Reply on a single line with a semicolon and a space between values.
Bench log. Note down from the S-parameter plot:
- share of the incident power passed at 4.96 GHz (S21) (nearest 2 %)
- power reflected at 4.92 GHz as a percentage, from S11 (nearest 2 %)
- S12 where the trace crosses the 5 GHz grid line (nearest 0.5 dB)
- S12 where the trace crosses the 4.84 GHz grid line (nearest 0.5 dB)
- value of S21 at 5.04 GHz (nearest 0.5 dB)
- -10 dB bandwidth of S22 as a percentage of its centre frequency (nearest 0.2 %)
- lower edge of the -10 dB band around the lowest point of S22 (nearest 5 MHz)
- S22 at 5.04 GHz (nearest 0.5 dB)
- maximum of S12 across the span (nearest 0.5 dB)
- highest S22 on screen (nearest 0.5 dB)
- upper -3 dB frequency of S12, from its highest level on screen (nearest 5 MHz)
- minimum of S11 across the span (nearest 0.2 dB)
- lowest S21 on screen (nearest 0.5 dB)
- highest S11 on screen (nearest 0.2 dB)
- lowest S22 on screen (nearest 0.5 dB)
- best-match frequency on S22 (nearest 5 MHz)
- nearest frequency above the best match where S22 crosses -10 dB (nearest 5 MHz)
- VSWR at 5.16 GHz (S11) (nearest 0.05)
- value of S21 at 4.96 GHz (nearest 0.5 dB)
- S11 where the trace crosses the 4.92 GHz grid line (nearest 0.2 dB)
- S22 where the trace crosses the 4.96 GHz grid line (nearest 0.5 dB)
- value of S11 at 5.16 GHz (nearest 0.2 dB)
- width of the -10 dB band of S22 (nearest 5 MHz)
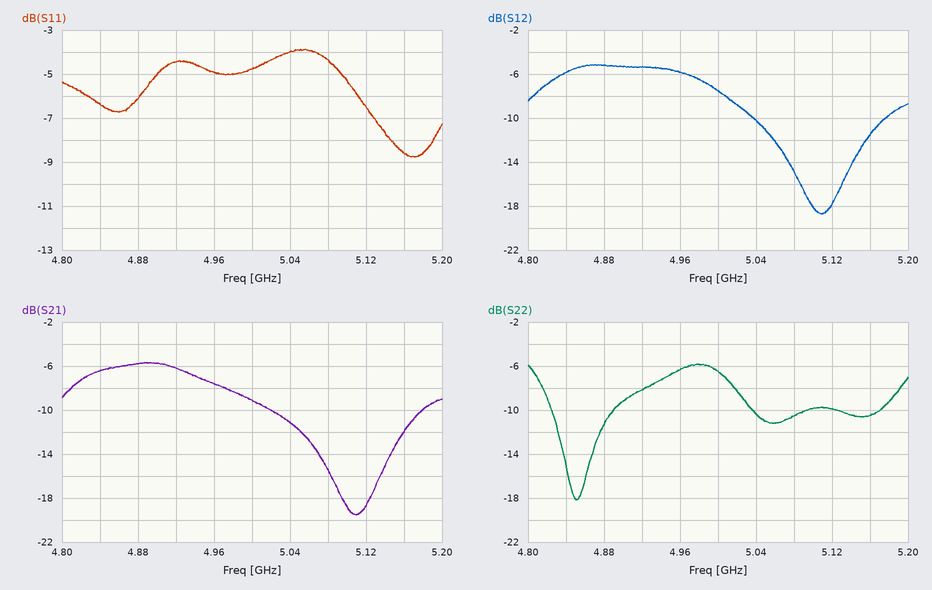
18 %; 36 %; -7.5 dB; -6.0 dB; -11.0 dB; 1.4 %; 4.825 GHz; -10.5 dB; -5.0 dB; -6.0 dB; 5.010 GHz; -8.8 dB; -19.5 dB; -3.8 dB; -18.0 dB; 4.850 GHz; 4.890 GHz; 2.20; -7.5 dB; -4.4 dB; -6.5 dB; -8.6 dB; 65 MHz
